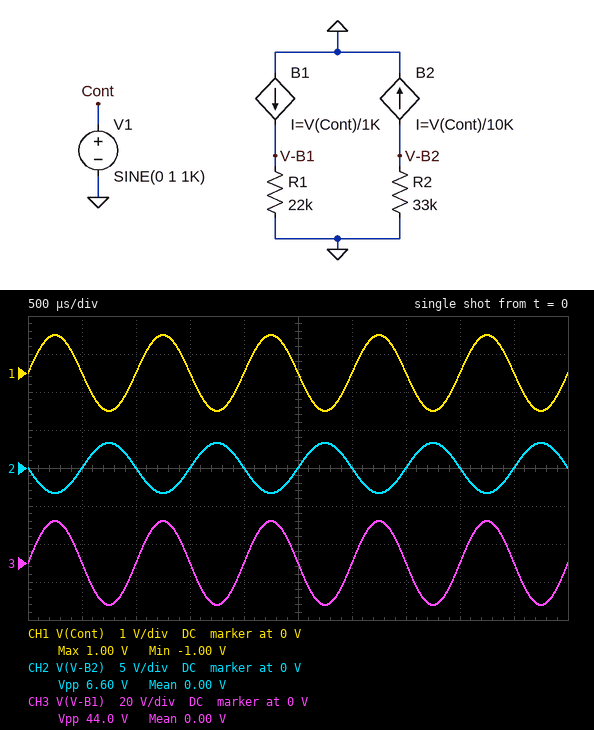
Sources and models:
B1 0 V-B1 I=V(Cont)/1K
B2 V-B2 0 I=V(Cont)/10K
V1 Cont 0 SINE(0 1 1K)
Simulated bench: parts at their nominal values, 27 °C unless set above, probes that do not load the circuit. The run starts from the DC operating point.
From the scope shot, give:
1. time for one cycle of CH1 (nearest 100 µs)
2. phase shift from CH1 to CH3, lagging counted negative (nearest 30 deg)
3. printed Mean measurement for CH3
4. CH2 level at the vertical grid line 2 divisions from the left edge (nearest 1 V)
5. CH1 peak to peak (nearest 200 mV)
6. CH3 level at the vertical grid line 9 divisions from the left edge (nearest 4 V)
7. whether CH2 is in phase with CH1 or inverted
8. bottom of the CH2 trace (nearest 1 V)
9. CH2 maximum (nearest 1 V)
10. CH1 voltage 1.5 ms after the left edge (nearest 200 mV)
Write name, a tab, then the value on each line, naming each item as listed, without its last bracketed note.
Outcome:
time for one cycle of CH1	1.0 ms
phase shift from CH1 to CH3, lagging counted negative	0 deg
printed Mean measurement for CH3	0.00 V
CH2 level at the vertical grid line 2 divisions from the left edge	0 V
CH1 peak to peak	2.0 V
CH3 level at the vertical grid line 9 divisions from the left edge	0 V
whether CH2 is in phase with CH1 or inverted	inverted
bottom of the CH2 trace	-3 V
CH2 maximum	3 V
CH1 voltage 1.5 ms after the left edge	0 V
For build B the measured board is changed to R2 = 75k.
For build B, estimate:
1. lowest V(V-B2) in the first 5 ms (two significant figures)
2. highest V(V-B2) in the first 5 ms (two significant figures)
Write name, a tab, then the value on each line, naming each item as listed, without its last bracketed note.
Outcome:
lowest V(V-B2) in the first 5 ms	-7.5 V
highest V(V-B2) in the first 5 ms	7.5 V
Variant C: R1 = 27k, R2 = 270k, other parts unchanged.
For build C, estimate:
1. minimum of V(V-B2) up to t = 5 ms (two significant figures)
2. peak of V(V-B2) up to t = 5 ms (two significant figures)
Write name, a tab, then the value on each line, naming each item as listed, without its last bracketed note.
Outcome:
minimum of V(V-B2) up to t = 5 ms	-27 V
peak of V(V-B2) up to t = 5 ms	27 V
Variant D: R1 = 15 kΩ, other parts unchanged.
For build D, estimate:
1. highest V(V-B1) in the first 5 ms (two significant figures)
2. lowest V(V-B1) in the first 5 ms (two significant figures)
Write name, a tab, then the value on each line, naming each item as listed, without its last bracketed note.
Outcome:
highest V(V-B1) in the first 5 ms	15 V
lowest V(V-B1) in the first 5 ms	-15 V
